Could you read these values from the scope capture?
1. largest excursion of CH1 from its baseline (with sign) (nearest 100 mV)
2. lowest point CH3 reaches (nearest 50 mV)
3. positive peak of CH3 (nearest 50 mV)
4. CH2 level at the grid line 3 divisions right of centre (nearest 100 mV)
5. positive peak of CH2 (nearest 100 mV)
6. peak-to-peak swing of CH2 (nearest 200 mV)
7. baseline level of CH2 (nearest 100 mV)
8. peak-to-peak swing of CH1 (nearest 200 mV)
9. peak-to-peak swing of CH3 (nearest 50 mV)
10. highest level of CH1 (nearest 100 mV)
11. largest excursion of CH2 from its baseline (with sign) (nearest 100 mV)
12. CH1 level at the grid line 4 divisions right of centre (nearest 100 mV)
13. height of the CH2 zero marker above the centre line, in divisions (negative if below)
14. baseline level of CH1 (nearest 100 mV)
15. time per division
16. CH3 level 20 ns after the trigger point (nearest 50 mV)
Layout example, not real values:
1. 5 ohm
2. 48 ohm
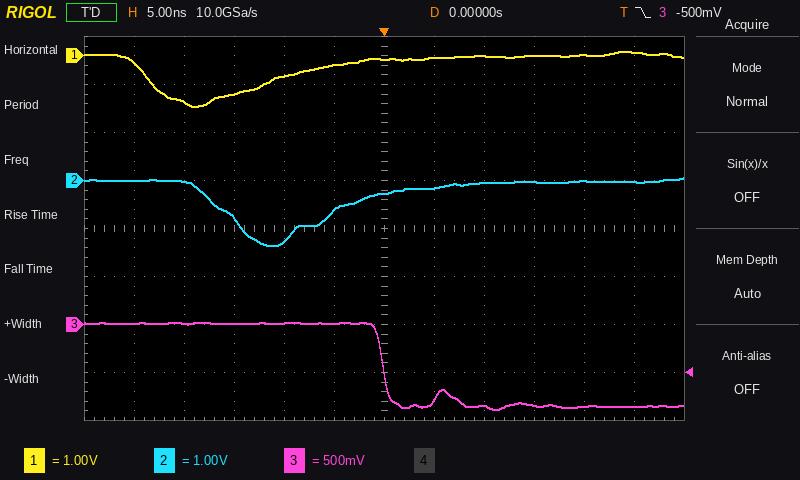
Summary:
1. -1.0 V
2. -900 mV
3. 0 mV
4. 0.0 V
5. 100 mV
6. 1.4 V
7. 0.0 V
8. 1.2 V
9. 900 mV
10. 100 mV
11. -1.3 V
12. 0.0 V
13. +1.0 div
14. 0.0 V
15. 5 ns
16. -850 mV
